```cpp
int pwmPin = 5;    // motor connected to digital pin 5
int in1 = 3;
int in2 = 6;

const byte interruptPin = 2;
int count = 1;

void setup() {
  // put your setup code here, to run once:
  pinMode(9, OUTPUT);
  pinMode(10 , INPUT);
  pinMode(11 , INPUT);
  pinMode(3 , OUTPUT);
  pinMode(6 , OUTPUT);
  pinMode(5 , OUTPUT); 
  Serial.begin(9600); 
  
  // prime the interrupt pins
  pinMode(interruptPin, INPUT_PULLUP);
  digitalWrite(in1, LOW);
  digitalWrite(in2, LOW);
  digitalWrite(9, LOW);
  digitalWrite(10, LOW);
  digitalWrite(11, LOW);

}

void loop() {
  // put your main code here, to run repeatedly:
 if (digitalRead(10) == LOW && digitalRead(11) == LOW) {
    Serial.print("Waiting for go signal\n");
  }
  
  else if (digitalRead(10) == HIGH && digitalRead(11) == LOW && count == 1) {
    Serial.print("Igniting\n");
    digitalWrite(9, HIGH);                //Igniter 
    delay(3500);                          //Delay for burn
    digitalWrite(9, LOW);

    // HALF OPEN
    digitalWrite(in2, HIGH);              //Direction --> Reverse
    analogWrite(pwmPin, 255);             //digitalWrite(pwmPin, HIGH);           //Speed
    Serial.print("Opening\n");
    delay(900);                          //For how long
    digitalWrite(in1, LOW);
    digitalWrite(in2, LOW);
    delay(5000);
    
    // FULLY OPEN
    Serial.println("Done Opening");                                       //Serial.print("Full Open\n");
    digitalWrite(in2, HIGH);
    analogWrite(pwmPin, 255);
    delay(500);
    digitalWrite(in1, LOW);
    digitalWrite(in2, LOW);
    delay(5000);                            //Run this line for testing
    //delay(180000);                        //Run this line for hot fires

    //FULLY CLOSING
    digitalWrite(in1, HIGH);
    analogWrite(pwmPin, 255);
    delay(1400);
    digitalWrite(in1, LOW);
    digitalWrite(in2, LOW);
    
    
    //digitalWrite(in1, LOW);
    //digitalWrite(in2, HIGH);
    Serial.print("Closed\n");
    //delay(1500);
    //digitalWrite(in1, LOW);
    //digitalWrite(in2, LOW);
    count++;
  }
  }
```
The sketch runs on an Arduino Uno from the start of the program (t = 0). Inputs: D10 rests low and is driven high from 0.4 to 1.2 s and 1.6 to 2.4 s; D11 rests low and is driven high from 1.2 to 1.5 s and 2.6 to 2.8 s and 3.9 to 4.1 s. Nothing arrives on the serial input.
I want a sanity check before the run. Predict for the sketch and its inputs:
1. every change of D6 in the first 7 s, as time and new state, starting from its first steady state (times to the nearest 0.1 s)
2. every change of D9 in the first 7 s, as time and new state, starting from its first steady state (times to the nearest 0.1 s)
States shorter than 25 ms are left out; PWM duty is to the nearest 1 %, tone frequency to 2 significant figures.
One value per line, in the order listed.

0 s low; 3.9 s high; 4.8 s low
0 s low; 0.4 s high; 3.9 s low
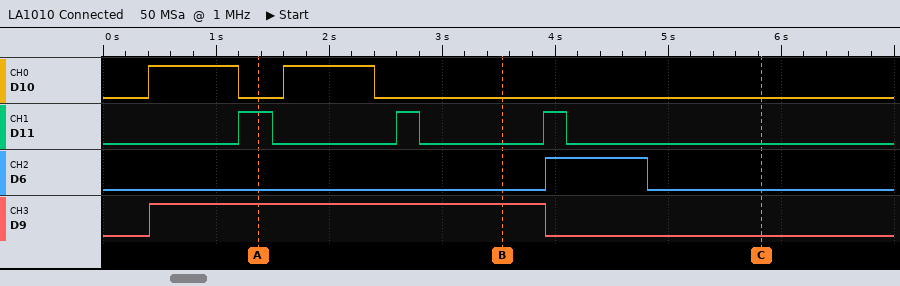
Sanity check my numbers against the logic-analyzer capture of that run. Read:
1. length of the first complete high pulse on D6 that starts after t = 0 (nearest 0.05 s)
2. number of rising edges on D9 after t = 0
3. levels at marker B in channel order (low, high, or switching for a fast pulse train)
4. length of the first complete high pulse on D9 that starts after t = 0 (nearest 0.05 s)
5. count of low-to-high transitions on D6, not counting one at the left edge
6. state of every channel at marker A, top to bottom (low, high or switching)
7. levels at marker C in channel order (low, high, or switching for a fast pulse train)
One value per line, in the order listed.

0.90 s
1
D10 low, D11 low, D6 low, D9 high
3.50 s
1
D10 low, D11 high, D6 low, D9 high
D10 low, D11 low, D6 low, D9 low
